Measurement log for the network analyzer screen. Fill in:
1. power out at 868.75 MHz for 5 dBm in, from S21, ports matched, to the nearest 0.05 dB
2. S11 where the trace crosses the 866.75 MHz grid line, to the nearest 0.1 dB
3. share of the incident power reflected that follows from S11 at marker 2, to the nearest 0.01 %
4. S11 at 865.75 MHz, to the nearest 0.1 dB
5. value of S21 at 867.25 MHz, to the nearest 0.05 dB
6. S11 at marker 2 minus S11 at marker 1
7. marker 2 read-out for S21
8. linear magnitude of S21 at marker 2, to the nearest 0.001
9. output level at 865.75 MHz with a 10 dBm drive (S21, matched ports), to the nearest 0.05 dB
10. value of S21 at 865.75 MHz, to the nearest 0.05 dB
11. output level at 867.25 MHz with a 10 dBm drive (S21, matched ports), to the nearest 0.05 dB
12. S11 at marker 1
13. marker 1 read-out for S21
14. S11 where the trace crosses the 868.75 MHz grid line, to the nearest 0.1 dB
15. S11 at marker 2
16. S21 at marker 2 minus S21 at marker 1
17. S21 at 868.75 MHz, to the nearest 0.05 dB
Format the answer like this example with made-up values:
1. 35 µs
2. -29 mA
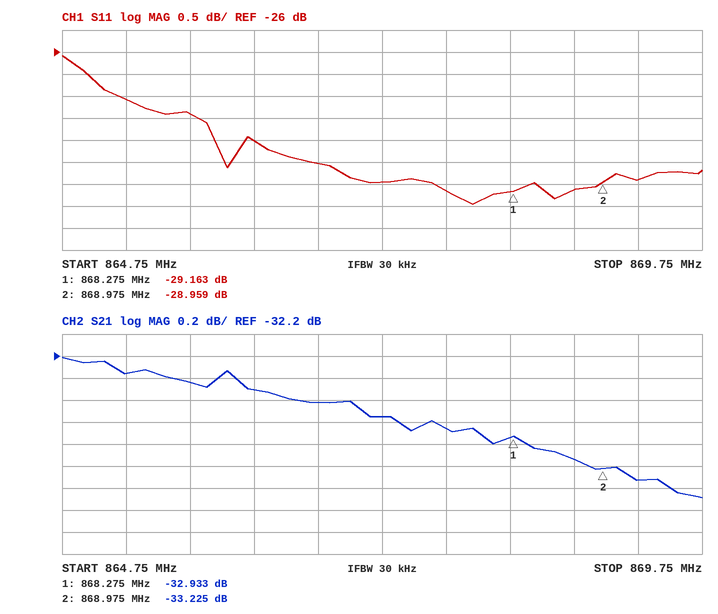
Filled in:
1. -28.15 dBm
2. -28.5 dB
3. 0.13 %
4. -27.4 dB
5. -32.75 dB
6. 0.204 dB
7. -33.225 dB
8. 0.022
9. -22.45 dBm
10. -32.45 dB
11. -22.75 dBm
12. -29.163 dB
13. -32.933 dB
14. -29.1 dB
15. -28.959 dB
16. -0.292 dB
17. -33.15 dB
